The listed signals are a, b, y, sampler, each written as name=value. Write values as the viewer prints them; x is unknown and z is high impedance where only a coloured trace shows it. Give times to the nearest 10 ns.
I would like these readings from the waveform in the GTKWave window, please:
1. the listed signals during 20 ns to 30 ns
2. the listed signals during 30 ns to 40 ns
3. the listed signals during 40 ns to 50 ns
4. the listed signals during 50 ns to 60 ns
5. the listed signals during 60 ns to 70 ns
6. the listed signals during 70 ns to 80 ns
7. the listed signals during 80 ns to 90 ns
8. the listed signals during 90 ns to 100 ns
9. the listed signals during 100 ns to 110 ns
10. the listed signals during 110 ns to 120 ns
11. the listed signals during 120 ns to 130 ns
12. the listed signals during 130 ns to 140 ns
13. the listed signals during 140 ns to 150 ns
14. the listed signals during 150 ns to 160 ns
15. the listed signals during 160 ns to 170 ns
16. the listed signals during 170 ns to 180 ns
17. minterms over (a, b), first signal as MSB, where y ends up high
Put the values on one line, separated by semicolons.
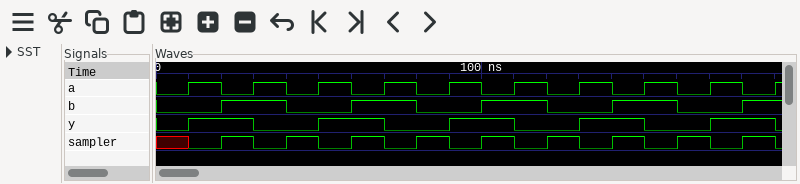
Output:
a=0, b=1, y=1, sampler=1; a=1, b=1, y=0, sampler=0; a=0, b=0, y=0, sampler=1; a=1, b=0, y=1, sampler=0; a=0, b=1, y=1, sampler=1; a=1, b=1, y=0, sampler=0; a=0, b=0, y=0, sampler=1; a=1, b=0, y=1, sampler=0; a=0, b=1, y=1, sampler=1; a=1, b=1, y=0, sampler=0; a=0, b=0, y=0, sampler=1; a=1, b=0, y=1, sampler=0; a=0, b=1, y=1, sampler=1; a=1, b=1, y=0, sampler=0; a=0, b=0, y=0, sampler=1; a=1, b=0, y=1, sampler=0; 1, 2
